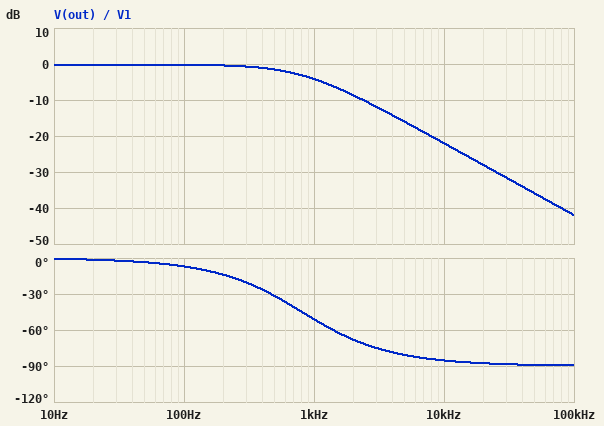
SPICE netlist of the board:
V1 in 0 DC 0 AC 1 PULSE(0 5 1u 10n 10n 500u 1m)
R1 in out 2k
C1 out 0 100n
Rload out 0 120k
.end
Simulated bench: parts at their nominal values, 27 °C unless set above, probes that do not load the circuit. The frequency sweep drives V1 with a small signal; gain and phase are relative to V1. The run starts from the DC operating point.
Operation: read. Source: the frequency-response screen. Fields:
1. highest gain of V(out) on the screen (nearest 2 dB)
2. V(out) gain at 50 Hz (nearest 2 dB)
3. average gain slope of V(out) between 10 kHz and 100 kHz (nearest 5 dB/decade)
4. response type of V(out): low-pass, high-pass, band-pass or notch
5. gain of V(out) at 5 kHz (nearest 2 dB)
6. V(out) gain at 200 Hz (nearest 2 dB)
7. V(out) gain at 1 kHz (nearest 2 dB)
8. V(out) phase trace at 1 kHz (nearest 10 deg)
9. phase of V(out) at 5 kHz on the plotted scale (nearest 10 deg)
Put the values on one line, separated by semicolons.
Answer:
0 dB; 0 dB; -20 dB/decade; low-pass; -16 dB; 0 dB; -4 dB; -50 deg; -80 deg
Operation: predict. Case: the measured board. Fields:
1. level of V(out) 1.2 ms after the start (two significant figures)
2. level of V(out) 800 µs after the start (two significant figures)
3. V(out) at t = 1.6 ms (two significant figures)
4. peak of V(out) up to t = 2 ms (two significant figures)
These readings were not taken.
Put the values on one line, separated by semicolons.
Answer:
3.3 V; 990 mV; 2.8 V; 4.6 V
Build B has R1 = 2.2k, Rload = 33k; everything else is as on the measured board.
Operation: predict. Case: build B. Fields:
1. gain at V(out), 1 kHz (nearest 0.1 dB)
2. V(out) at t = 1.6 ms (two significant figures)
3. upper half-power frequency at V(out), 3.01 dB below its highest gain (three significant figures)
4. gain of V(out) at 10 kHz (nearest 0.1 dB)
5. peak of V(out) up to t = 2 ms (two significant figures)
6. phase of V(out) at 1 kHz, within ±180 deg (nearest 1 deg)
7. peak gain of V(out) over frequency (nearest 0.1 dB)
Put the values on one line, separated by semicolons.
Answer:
-4.8 dB; 2.7 V; 772 Hz; -22.8 dB; 4.3 V; -52 deg; -0.6 dB
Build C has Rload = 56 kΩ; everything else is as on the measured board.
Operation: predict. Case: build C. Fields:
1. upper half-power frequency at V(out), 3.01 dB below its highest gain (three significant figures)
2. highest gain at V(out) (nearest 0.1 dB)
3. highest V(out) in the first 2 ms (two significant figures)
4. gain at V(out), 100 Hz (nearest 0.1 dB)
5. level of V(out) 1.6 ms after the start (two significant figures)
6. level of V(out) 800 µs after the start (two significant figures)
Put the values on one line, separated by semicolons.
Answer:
824 Hz; -0.3 dB; 4.5 V; -0.4 dB; 2.7 V; 950 mV
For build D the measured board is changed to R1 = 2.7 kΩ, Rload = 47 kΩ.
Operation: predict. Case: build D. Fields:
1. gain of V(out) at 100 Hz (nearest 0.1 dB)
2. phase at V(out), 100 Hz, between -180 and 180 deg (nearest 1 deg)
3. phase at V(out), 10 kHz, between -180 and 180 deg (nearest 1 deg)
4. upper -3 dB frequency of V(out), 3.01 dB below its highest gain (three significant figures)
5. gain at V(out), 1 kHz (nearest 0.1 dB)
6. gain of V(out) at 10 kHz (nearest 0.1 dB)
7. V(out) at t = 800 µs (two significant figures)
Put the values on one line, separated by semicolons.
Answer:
-0.6 dB; -9 deg; -86 deg; 623 Hz; -6.0 dB; -24.6 dB; 1.3 V
